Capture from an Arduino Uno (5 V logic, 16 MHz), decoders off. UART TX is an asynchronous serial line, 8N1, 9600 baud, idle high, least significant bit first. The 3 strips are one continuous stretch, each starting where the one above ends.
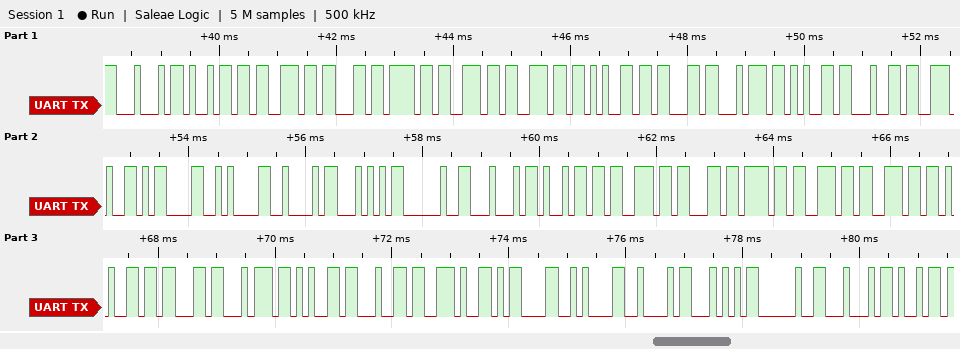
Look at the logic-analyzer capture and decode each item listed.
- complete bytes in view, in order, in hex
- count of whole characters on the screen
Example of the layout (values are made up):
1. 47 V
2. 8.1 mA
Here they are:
1. 44 69 73 63 6F 6E 6E 65 63 74 65 64 2E 0D 0A 42 54 20 44 69 73 63 6F 6E 6E 65 63 74 65 64 2E 0D 0A 42 54 20 44 69
2. 38
